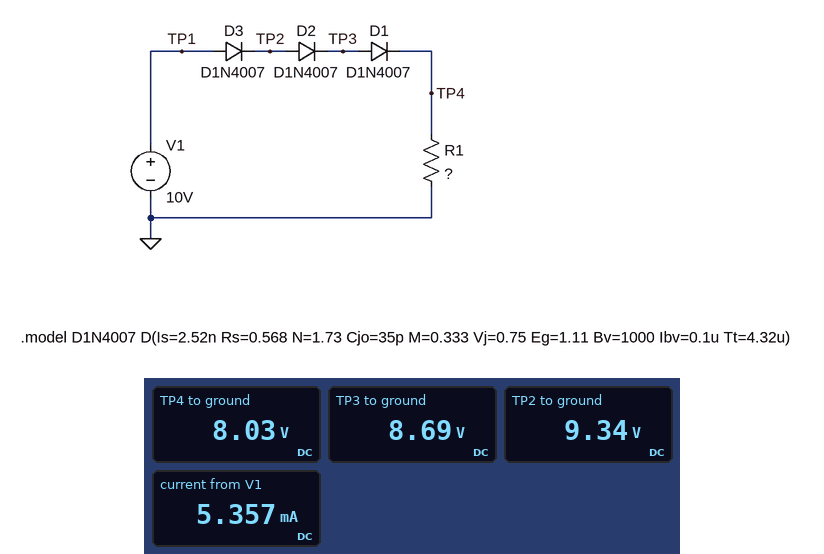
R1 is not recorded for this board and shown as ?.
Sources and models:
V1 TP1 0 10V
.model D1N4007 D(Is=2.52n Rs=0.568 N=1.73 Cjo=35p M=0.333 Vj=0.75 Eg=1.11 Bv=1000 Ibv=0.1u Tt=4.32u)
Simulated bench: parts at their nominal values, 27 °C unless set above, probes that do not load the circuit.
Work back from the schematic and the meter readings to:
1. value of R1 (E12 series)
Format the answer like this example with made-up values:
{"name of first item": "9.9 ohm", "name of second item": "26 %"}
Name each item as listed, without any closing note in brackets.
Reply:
{"value of R1": "1.5 kΩ"}
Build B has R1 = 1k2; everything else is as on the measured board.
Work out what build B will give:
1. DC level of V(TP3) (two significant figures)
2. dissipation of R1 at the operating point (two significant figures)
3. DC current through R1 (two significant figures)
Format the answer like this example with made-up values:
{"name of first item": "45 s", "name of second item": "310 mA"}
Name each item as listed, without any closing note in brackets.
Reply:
{"DC level of V(TP3)": "8.7 V", "dissipation of R1 at the operating point": "53 mW", "DC current through R1": "6.7 mA"}
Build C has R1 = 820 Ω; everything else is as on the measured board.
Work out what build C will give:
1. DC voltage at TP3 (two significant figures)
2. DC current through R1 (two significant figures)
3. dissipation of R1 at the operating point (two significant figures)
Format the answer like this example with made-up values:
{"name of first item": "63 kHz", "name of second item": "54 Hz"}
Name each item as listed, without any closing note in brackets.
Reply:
{"DC voltage at TP3": "8.6 V", "DC current through R1": "9.7 mA", "dissipation of R1 at the operating point": "77 mW"}
